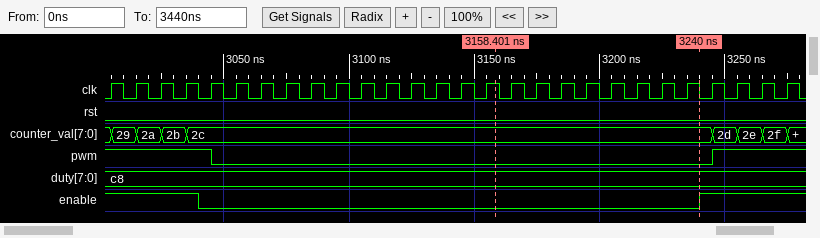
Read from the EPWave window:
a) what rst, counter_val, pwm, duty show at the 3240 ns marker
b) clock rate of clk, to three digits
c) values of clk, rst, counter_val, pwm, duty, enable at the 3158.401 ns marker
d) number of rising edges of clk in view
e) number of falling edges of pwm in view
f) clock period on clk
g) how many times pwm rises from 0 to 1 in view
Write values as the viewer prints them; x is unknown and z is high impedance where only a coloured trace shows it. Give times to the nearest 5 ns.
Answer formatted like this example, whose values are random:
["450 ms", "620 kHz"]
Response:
["rst=0, counter_val=2c, pwm=0, duty=c8", "100 MHz", "clk=1, rst=0, counter_val=2c, pwm=0, duty=c8, enable=0", "28", "1", "10 ns", "1"]
